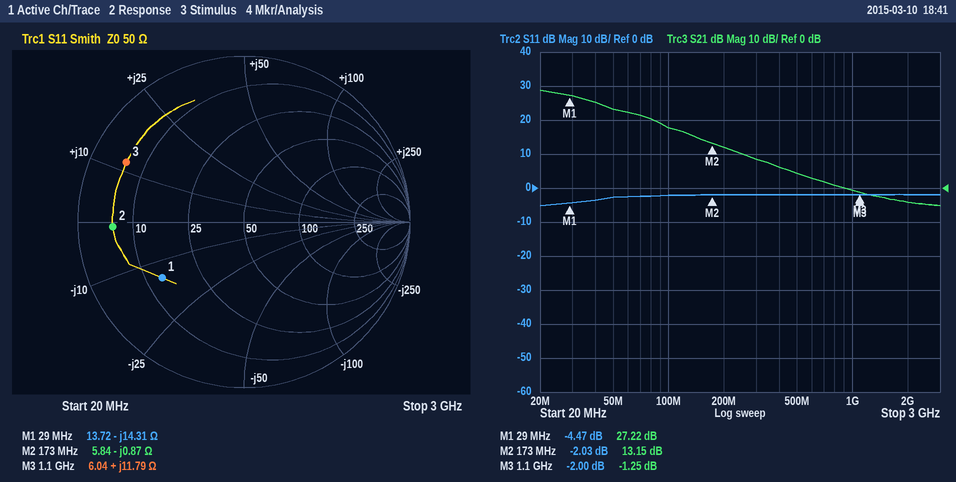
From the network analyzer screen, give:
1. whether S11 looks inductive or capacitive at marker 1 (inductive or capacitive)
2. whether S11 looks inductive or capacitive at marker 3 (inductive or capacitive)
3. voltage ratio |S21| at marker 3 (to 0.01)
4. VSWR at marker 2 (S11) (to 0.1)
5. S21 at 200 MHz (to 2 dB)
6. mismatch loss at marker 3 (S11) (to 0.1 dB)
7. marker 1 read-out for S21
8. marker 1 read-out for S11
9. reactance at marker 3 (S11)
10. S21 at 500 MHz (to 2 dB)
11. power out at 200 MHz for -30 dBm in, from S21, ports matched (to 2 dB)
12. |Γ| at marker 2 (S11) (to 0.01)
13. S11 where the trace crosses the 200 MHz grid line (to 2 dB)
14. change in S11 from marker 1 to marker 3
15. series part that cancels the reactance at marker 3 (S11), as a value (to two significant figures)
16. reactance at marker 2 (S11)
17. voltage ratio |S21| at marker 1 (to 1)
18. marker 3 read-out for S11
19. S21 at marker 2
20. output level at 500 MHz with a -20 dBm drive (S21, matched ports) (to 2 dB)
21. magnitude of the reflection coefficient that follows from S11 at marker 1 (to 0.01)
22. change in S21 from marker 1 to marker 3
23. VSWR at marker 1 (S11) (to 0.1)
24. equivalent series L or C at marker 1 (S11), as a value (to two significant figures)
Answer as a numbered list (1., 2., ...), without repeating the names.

1. capacitive
2. inductive
3. 0.87
4. 8.6
5. 12 dB
6. 4.3 dB
7. 27.22 dB
8. -4.47 dB
9. +11.79 Ω
10. 4 dB
11. -18 dBm
12. 0.79
13. -2 dB
14. 2.47 dB
15. 12 pF
16. -0.87 Ω
17. 23
18. -2.00 dB
19. 13.15 dB
20. -16 dBm
21. 0.60
22. -28.47 dB
23. 4.0
24. 380 pF
